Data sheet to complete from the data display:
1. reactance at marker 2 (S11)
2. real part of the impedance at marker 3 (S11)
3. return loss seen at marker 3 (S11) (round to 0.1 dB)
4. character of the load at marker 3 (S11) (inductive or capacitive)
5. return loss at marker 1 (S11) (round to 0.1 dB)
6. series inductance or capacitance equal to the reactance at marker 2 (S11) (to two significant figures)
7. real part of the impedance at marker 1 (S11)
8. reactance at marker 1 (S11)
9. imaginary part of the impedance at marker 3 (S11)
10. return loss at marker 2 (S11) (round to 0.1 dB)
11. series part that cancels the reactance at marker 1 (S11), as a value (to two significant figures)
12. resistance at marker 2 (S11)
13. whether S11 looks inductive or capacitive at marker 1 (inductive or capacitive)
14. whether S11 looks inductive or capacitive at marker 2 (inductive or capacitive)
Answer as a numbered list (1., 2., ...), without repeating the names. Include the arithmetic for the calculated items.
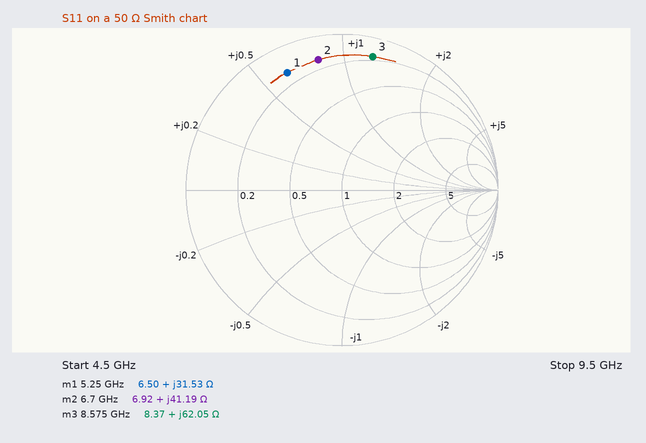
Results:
1. +41.19 Ω
2. 8.37 Ω
3. 1.1 dB
4. inductive
5. 1.6 dB
6. L = 41.19 Ω/(2π × 6.7 GHz) ≈ 978 pH, so 980 pH to two significant figures
7. 6.50 Ω
8. +31.53 Ω
9. +62.05 Ω
10. 1.4 dB
11. C = 1/(2π × 5.25 GHz × 31.53 Ω) ≈ 961 fF, so 960 fF to two significant figures
12. 6.92 Ω
13. inductive
14. inductive
